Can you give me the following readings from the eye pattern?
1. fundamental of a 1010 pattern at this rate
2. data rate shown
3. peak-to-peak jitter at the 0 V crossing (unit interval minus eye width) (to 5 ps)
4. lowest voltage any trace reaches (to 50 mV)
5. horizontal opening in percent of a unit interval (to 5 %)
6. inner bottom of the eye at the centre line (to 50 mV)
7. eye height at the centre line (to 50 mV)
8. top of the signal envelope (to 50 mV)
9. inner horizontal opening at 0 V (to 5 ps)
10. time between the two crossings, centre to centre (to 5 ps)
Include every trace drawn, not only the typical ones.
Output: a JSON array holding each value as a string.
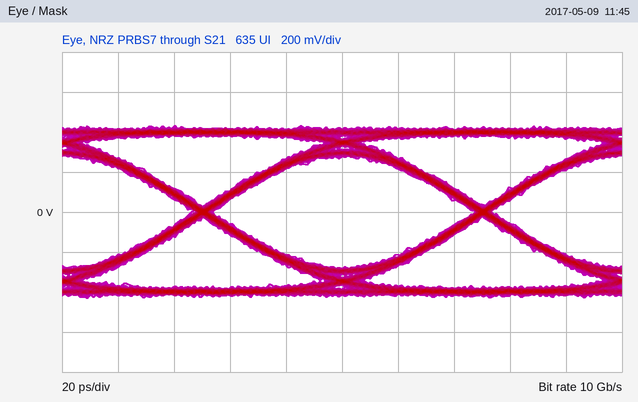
["5 GHz", "10 Gb/s", "5 ps", "-450 mV", "95 %", "-300 mV", "550 mV", "450 mV", "95 ps", "100 ps"]
